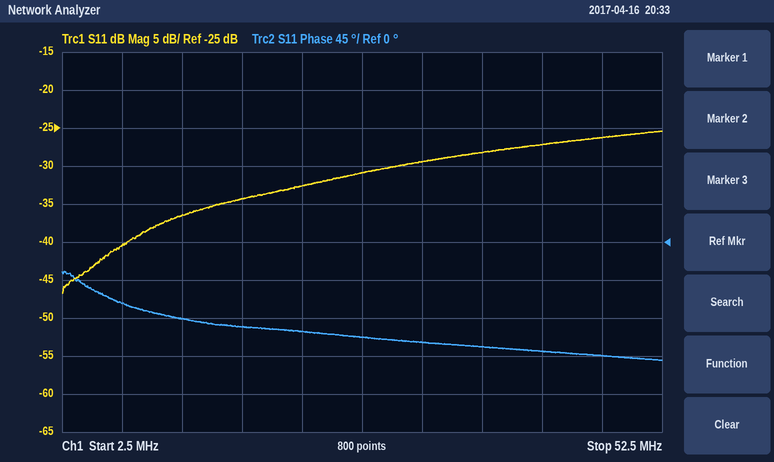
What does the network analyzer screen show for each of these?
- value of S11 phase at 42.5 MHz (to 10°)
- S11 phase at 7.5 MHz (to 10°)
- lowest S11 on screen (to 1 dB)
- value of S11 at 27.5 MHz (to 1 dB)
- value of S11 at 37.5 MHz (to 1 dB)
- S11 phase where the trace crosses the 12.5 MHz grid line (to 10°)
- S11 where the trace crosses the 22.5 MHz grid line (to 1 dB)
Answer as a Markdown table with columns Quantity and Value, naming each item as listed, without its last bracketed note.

| Quantity | Value |
|---|---|
| value of S11 phase at 42.5 MHz | -130° |
| S11 phase at 7.5 MHz | -70° |
| lowest S11 on screen | -47 dB |
| value of S11 at 27.5 MHz | -31 dB |
| value of S11 at 37.5 MHz | -28 dB |
| S11 phase where the trace crosses the 12.5 MHz grid line | -90° |
| S11 where the trace crosses the 22.5 MHz grid line | -33 dB |
